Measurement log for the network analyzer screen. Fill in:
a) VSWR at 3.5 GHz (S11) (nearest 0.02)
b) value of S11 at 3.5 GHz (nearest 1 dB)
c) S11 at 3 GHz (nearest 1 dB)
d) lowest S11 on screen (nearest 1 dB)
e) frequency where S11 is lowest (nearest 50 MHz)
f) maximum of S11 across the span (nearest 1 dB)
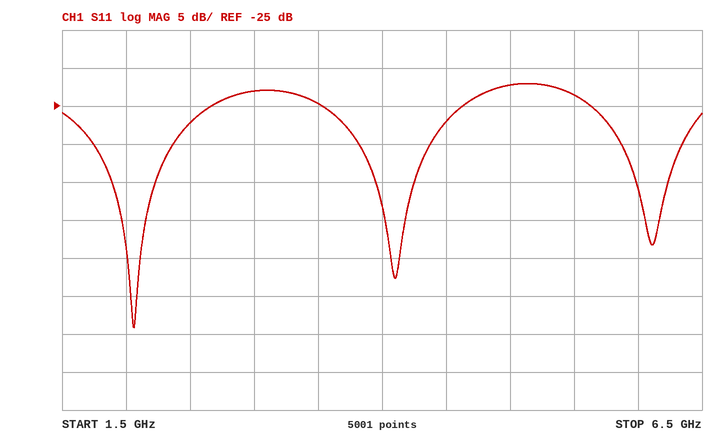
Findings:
1.12
-25 dB
-23 dB
-54 dB
2.05 GHz
-22 dB
